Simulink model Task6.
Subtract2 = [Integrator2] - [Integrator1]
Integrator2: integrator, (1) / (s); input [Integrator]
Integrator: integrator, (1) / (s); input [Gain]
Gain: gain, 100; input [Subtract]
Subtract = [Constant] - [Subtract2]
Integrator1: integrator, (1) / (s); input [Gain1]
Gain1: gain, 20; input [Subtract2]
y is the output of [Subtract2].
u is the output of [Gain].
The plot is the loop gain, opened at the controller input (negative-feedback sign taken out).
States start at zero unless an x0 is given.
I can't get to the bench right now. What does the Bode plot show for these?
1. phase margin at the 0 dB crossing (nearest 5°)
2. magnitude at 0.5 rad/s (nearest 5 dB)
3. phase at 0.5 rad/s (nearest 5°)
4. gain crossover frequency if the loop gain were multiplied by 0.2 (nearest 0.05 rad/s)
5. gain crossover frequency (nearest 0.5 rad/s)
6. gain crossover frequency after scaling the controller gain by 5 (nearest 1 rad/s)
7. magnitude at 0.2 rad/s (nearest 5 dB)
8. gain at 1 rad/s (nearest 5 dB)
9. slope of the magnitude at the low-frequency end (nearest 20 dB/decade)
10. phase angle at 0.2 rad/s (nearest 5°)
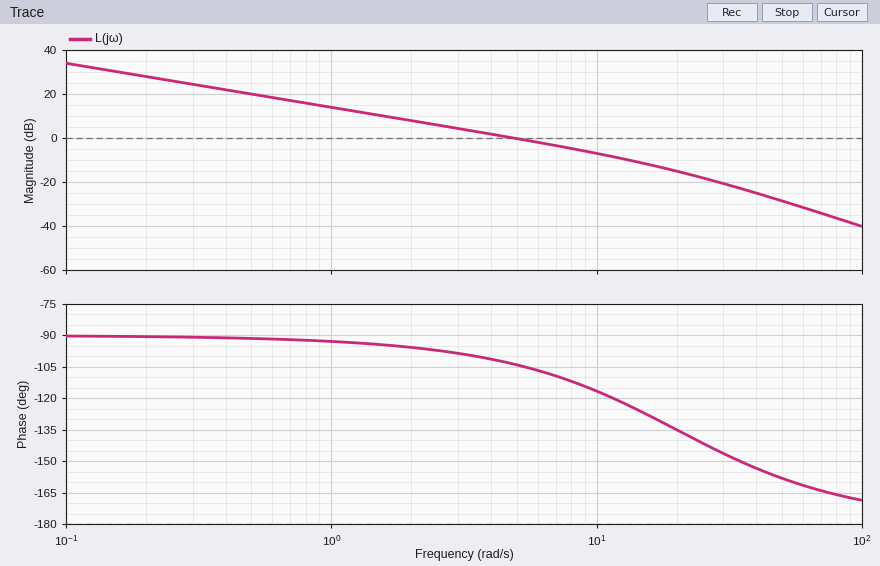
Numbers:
75°
20 dB
-90°
1.00 rad/s
5.0 rad/s
18 rad/s
30 dB
15 dB
-20 dB/decade
-90°
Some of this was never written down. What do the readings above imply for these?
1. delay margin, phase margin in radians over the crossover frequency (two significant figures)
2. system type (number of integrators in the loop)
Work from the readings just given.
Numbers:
0.26 s
1
